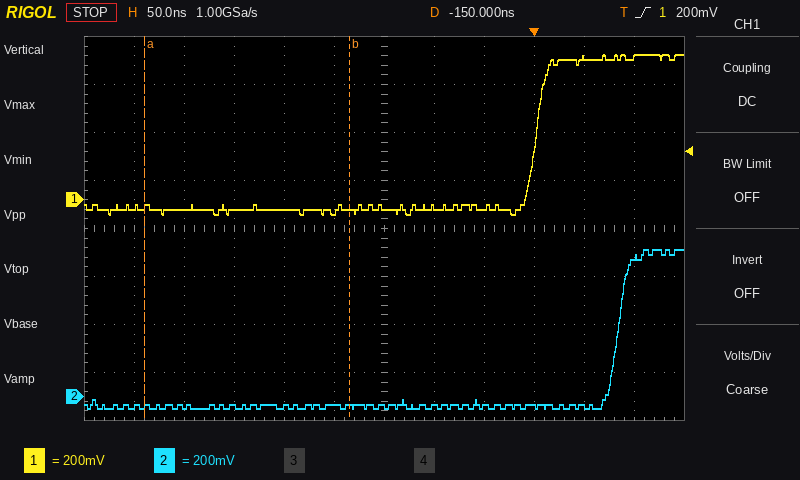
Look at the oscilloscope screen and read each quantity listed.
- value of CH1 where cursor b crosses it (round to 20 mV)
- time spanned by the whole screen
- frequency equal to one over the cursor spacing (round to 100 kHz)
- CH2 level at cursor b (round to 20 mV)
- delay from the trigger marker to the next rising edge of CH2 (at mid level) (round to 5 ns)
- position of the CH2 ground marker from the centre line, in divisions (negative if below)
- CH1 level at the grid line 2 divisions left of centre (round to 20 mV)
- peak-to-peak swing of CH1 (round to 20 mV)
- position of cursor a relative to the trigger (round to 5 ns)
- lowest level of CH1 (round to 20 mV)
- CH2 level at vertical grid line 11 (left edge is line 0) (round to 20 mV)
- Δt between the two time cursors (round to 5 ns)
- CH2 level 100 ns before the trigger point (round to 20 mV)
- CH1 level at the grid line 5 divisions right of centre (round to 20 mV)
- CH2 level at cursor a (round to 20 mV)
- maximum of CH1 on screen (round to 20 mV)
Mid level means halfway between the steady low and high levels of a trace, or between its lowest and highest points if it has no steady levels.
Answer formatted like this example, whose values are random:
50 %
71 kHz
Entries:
-40 mV
600 ns
4.9 MHz
-40 mV
85 ns
-3.5 div
-40 mV
660 mV
-390 ns
-60 mV
580 mV
205 ns
-40 mV
600 mV
-40 mV
600 mV
